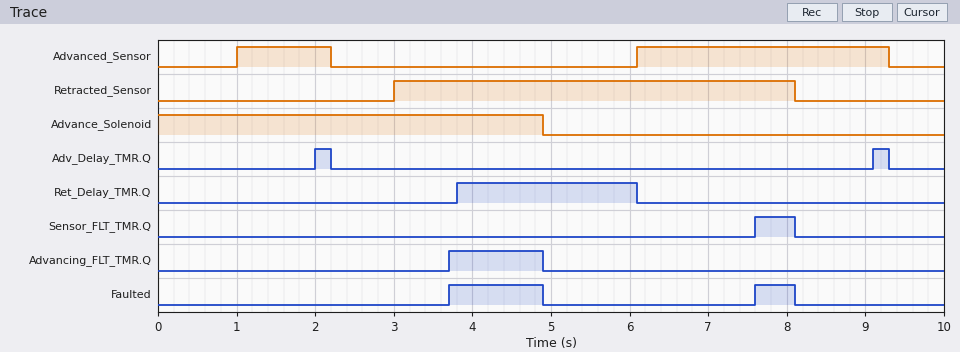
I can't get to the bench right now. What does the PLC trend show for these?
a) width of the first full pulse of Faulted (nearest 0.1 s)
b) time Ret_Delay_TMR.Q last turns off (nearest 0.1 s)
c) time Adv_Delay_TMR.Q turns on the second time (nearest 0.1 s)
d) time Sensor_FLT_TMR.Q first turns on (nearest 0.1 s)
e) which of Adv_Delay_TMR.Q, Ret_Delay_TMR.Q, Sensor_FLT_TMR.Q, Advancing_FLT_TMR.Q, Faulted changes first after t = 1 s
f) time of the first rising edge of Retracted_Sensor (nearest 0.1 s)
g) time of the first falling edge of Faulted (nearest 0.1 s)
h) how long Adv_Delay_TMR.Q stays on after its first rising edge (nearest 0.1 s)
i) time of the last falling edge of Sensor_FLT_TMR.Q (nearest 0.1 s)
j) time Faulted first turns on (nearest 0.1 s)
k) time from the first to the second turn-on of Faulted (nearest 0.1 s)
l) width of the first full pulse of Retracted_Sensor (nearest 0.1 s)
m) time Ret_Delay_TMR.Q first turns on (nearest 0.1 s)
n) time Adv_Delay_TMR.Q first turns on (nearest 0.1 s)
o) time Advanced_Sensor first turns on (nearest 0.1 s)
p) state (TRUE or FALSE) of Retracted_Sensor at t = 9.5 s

1.2 s
6.1 s
9.1 s
7.6 s
Adv_Delay_TMR.Q
3.0 s
4.9 s
0.2 s
8.1 s
3.7 s
3.9 s
5.1 s
3.8 s
2.0 s
1.0 s
FALSE
